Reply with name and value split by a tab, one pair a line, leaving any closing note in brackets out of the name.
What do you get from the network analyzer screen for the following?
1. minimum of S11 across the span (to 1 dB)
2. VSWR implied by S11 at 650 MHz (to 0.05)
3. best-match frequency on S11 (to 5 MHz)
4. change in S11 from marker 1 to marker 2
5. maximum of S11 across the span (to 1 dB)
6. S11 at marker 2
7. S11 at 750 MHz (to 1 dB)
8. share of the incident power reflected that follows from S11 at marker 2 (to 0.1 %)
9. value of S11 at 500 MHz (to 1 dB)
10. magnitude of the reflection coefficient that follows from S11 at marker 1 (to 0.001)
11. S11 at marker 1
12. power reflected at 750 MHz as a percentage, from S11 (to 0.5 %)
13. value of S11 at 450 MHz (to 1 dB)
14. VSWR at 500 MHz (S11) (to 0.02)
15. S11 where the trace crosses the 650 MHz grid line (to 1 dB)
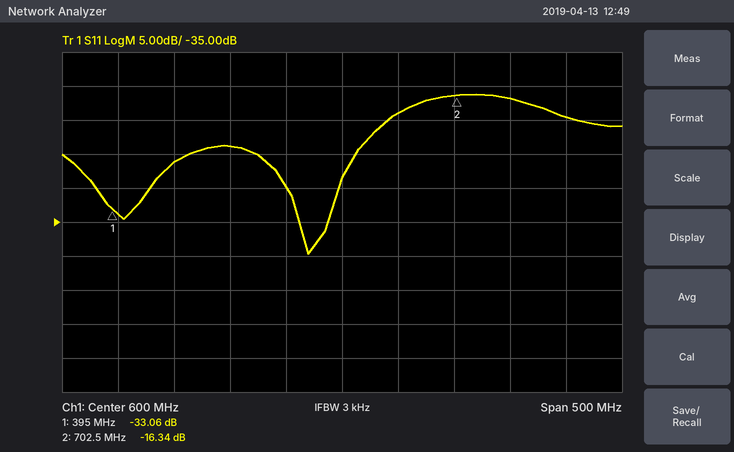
minimum of S11 across the span	-40 dB
VSWR implied by S11 at 650 MHz	1.25
best-match frequency on S11	570 MHz
change in S11 from marker 1 to marker 2	16.72 dB
maximum of S11 across the span	-16 dB
S11 at marker 2	-16.34 dB
S11 at 750 MHz	-17 dB
share of the incident power reflected that follows from S11 at marker 2	2.3 %
value of S11 at 500 MHz	-24 dB
magnitude of the reflection coefficient that follows from S11 at marker 1	0.022
S11 at marker 1	-33.06 dB
power reflected at 750 MHz as a percentage, from S11	2.0 %
value of S11 at 450 MHz	-26 dB
VSWR at 500 MHz (S11)	1.14
S11 where the trace crosses the 650 MHz grid line	-19 dB
